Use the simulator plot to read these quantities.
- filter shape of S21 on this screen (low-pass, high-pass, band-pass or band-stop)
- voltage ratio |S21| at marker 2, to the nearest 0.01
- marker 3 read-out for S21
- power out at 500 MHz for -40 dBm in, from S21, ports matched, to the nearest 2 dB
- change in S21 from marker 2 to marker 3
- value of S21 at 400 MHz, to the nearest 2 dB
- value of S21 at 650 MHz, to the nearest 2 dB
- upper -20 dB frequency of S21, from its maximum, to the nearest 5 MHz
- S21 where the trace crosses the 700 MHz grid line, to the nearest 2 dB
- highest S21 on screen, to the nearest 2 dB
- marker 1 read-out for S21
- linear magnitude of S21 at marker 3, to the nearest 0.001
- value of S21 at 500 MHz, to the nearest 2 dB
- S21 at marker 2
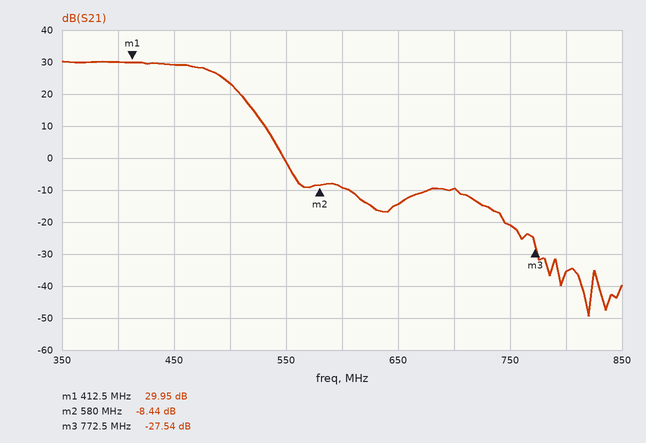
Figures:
low-pass
0.38
-27.54 dB
-16 dBm
-19.10 dB
30 dB
-14 dB
530 MHz
-10 dB
30 dB
29.95 dB
0.042
24 dB
-8.44 dB
